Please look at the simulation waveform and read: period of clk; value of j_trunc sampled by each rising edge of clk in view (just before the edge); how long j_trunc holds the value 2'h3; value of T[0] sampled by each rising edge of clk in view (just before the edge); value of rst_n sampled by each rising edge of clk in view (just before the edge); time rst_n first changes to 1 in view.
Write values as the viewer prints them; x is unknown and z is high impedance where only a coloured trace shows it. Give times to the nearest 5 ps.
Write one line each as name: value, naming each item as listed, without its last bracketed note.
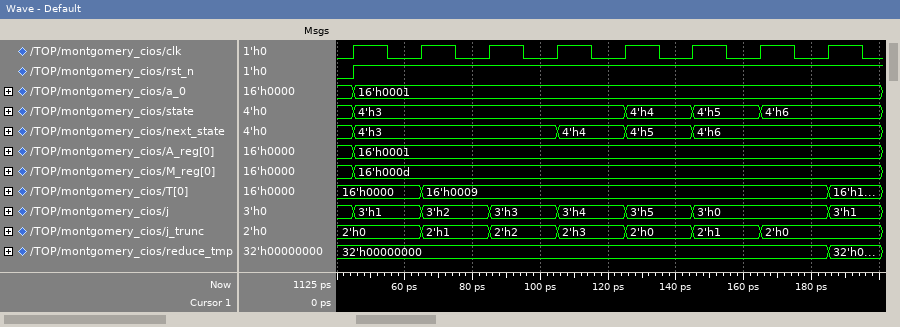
period of clk: 20 ps
value of j_trunc sampled by each rising edge of clk in view: 2'h0, 2'h0, 2'h1, 2'h2, 2'h3, 2'h0, 2'h1, 2'h0
how long j_trunc holds the value 2'h3: 20 ps
value of T[0] sampled by each rising edge of clk in view: 16'h0000, 16'h0000, 16'h0009, 16'h0009, 16'h0009, 16'h0009, 16'h0009, 16'h0009
value of rst_n sampled by each rising edge of clk in view: 0 1 1 1 1 1 1 1
time rst_n first changes to 1 in view: 45 ps
